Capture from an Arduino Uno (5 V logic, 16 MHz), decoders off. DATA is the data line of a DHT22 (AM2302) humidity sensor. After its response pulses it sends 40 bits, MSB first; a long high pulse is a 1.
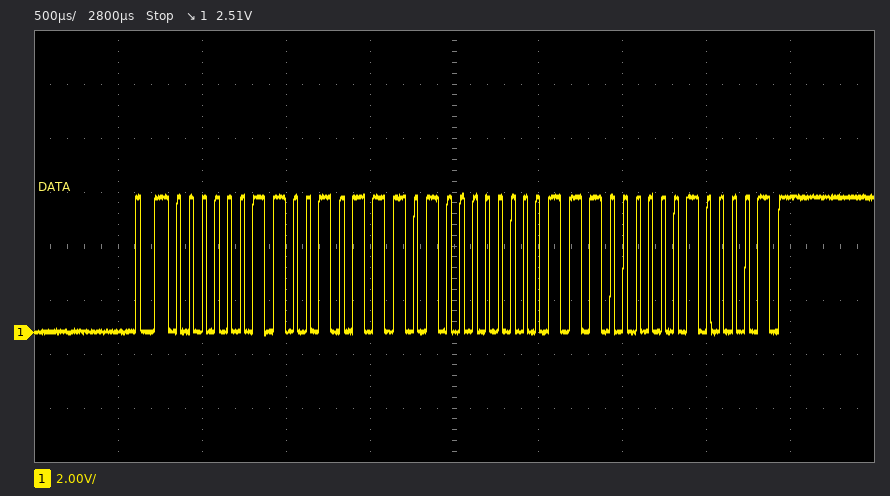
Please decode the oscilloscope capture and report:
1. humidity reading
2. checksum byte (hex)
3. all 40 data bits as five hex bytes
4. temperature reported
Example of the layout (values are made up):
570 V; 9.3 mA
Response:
81.4 %; 0x21; 03 2E 80 70 21; -11.2 °C
